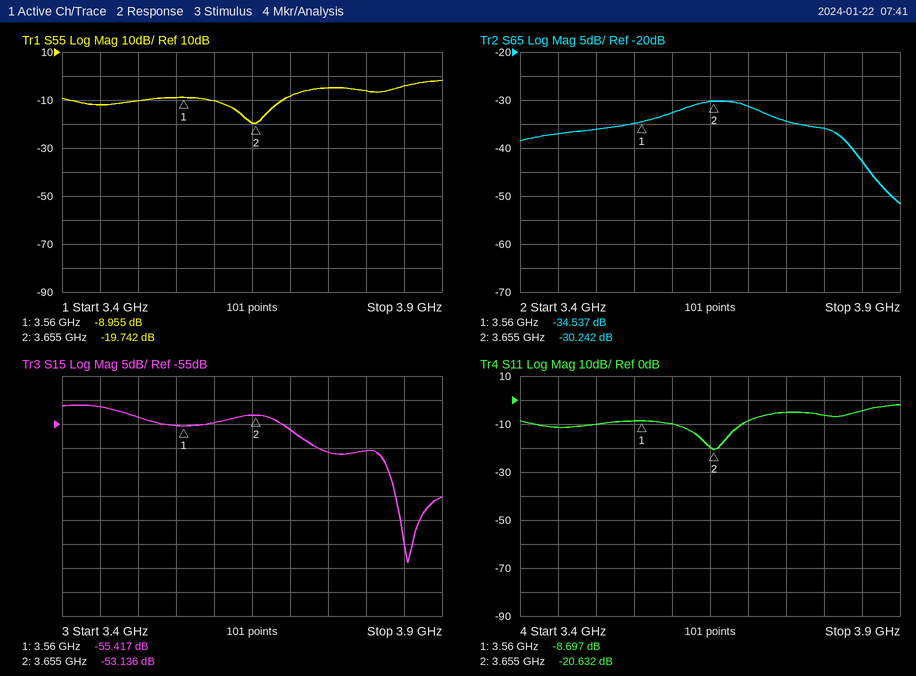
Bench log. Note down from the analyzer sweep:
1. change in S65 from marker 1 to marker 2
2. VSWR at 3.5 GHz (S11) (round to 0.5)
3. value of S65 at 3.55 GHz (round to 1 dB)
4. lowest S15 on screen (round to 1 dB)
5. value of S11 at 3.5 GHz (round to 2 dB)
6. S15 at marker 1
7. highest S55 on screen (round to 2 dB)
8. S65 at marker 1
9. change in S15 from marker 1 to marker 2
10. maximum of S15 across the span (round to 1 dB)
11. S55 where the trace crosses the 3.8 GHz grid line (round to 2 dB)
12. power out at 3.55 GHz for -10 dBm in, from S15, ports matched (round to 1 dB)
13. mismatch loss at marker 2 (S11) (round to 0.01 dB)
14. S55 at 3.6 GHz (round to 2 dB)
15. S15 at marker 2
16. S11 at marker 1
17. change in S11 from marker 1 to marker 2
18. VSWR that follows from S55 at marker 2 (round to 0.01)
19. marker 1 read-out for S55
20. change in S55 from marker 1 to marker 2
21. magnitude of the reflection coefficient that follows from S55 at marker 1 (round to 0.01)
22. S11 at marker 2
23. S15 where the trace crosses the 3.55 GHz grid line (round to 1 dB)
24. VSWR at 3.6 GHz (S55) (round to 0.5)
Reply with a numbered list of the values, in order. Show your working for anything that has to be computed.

1. -30.242 − (-34.537) = 4.295 dB
2. |Γ| = 10^(-10/20) = 0.3162; VSWR = (1 + 0.3162)/(1 − 0.3162) ≈ 1.92, so 2.0 to the nearest 0.5
3. -35 dB
4. -84 dB
5. -10 dB
6. -55.417 dB
7. -2 dB
8. -34.537 dB
9. -53.136 − (-55.417) = 2.281 dB
10. -51 dB
11. -6 dB
12. -10 dBm + (-55 dB) = -65 dBm
13. −10 log10(1 − 10^(-20.632/10)) ≈ 0.04 dB
14. -10 dB
15. -53.136 dB
16. -8.697 dB
17. -20.632 − (-8.697) = -11.935 dB
18. (1 + 0.1030)/(1 − 0.1030) ≈ 1.23
19. -8.955 dB
20. -19.742 − (-8.955) = -10.787 dB
21. 10^(-8.955/20) ≈ 0.36
22. -20.632 dB
23. -55 dB
24. |Γ| = 10^(-10/20) = 0.3162; VSWR = (1 + 0.3162)/(1 − 0.3162) ≈ 1.92, so 2.0 to the nearest 0.5
